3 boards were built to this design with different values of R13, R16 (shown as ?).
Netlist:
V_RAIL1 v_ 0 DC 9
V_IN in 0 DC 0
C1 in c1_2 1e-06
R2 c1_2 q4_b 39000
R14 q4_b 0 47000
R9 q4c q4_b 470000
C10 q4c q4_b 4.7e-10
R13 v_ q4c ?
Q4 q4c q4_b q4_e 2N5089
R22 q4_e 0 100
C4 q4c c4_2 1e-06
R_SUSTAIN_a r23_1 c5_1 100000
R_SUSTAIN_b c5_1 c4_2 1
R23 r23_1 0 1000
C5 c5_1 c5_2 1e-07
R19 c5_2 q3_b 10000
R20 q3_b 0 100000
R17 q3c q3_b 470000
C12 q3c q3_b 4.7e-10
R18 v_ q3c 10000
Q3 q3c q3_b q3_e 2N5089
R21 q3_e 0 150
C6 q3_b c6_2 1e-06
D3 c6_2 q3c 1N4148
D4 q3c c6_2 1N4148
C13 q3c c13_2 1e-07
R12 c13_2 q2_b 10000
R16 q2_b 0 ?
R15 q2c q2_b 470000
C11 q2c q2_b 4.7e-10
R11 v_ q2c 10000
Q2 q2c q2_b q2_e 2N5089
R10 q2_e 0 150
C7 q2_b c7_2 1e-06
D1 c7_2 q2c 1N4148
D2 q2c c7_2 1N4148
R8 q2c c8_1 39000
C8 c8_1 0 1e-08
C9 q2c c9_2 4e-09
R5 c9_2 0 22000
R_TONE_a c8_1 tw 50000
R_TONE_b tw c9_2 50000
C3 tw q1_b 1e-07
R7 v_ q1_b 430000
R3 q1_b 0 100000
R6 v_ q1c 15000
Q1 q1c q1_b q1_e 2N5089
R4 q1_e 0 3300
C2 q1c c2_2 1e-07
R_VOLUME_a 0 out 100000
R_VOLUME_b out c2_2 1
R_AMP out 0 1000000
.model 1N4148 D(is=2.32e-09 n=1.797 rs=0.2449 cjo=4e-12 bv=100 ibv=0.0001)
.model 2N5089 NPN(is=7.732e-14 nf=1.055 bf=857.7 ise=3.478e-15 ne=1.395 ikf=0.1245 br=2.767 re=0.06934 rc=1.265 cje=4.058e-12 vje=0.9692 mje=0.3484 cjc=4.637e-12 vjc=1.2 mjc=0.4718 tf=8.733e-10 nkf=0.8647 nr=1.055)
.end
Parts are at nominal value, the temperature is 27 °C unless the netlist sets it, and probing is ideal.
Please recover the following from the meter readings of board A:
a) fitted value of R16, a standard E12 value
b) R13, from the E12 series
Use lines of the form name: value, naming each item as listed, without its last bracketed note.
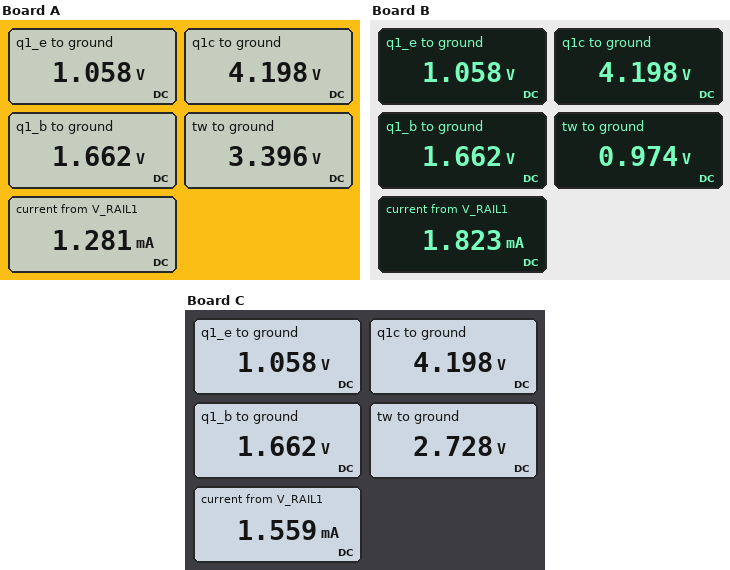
fitted value of R16, a standard E12 value: 39 kΩ
R13, from the E12 series: 5.6 kΩ
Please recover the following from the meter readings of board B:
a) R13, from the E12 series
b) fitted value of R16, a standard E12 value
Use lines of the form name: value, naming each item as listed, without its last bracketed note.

R13, from the E12 series: 5.6 kΩ
fitted value of R16, a standard E12 value: 330 kΩ
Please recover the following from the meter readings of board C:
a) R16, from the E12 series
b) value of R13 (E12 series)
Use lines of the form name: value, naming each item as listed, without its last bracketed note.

R16, from the E12 series: 56 kΩ
value of R13: 3.3 kΩ
